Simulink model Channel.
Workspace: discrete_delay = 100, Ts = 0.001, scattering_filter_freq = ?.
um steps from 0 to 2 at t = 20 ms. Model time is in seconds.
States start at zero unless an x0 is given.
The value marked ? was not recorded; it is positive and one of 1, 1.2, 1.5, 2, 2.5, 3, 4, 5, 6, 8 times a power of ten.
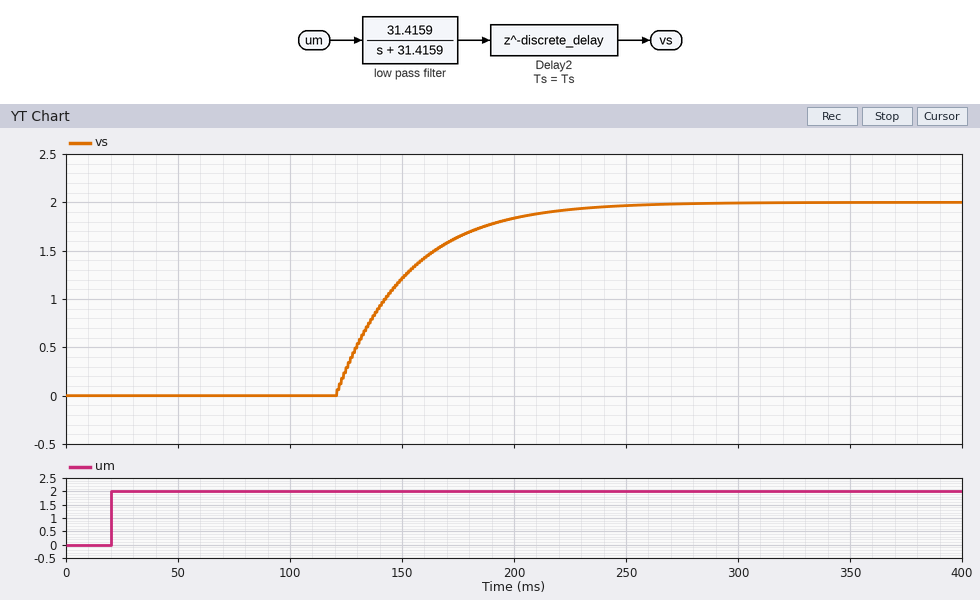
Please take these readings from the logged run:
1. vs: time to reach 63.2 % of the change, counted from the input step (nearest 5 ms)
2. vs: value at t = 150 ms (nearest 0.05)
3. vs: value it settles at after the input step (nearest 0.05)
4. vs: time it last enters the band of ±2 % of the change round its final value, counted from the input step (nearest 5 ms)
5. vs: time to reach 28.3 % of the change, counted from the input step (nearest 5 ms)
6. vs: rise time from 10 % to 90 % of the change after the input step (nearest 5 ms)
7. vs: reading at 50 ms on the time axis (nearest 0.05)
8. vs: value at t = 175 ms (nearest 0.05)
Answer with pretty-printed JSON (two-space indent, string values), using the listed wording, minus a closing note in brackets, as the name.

{
  "vs: time to reach 63.2 % of the change, counted from the input step": "130 ms",
  "vs: value at t = 150 ms": "1.20",
  "vs: value it settles at after the input step": "2.00",
  "vs: time it last enters the band of ±2 % of the change round its final value, counted from the input step": "225 ms",
  "vs: time to reach 28.3 % of the change, counted from the input step": "110 ms",
  "vs: rise time from 10 % to 90 % of the change after the input step": "70 ms",
  "vs: reading at 50 ms on the time axis": "0.00",
  "vs: value at t = 175 ms": "1.65"
}
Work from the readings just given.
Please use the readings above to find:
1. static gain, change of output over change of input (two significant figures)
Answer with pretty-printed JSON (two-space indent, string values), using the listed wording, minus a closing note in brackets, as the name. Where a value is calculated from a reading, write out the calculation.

{
  "static gain, change of output over change of input": "(2 - 0) / (2 - 0) = 1.0"
}
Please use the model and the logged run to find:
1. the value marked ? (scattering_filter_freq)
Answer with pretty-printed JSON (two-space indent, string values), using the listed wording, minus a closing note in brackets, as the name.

{
  "the value marked ?": "5"
}
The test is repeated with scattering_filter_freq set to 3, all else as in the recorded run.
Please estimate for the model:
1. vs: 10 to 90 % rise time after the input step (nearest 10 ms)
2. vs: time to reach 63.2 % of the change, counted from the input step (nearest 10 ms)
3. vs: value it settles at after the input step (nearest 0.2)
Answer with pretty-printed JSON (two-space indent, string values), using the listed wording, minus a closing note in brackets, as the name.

{
  "vs: 10 to 90 % rise time after the input step": "120 ms",
  "vs: time to reach 63.2 % of the change, counted from the input step": "150 ms",
  "vs: value it settles at after the input step": "2.0"
}
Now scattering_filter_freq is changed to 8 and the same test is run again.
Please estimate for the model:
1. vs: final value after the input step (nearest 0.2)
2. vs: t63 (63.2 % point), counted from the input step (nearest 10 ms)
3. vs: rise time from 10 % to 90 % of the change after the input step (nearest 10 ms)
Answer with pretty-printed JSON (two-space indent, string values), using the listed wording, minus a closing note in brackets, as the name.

{
  "vs: final value after the input step": "2.0",
  "vs: t63 (63.2 % point), counted from the input step": "120 ms",
  "vs: rise time from 10 % to 90 % of the change after the input step": "40 ms"
}
